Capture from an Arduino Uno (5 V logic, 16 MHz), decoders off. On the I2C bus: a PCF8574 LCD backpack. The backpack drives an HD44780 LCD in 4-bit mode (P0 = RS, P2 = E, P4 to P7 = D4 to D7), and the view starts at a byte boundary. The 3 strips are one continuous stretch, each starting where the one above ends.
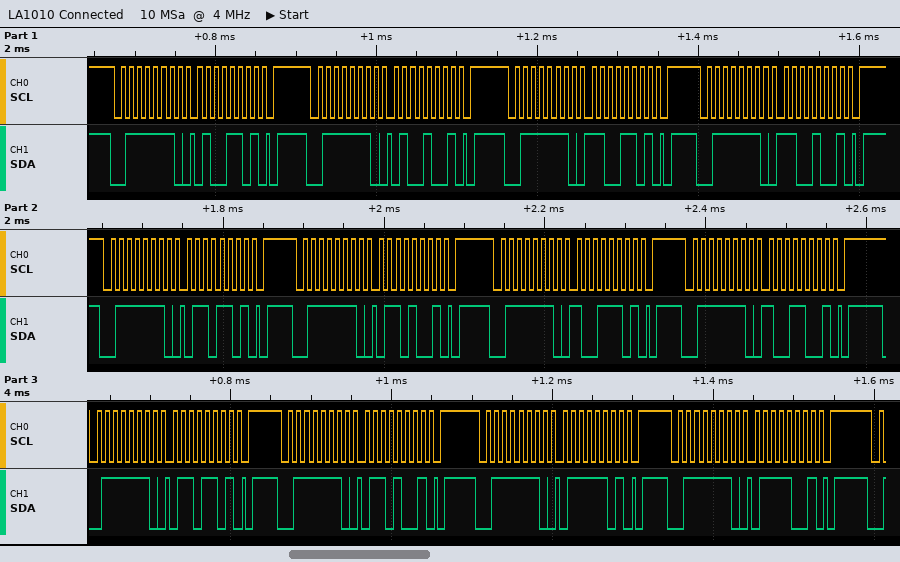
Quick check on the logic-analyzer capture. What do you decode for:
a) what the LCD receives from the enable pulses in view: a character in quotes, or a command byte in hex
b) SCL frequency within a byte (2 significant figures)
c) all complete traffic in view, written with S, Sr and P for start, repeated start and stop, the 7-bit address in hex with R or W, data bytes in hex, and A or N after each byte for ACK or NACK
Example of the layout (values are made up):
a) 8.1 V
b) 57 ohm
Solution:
a) 'L' 'i' 'g'
b) 100 kHz
c) S 3FW A 4D A P S 3FW A 49 A P S 3FW A CD A P S 3FW A C9 A P S 3FW A 6D A P S 3FW A 69 A P S 3FW A 9D A P S 3FW A 99 A P S 3FW A 6D A P S 3FW A 69 A P S 3FW A 7D A P S 3FW A 79 A P
